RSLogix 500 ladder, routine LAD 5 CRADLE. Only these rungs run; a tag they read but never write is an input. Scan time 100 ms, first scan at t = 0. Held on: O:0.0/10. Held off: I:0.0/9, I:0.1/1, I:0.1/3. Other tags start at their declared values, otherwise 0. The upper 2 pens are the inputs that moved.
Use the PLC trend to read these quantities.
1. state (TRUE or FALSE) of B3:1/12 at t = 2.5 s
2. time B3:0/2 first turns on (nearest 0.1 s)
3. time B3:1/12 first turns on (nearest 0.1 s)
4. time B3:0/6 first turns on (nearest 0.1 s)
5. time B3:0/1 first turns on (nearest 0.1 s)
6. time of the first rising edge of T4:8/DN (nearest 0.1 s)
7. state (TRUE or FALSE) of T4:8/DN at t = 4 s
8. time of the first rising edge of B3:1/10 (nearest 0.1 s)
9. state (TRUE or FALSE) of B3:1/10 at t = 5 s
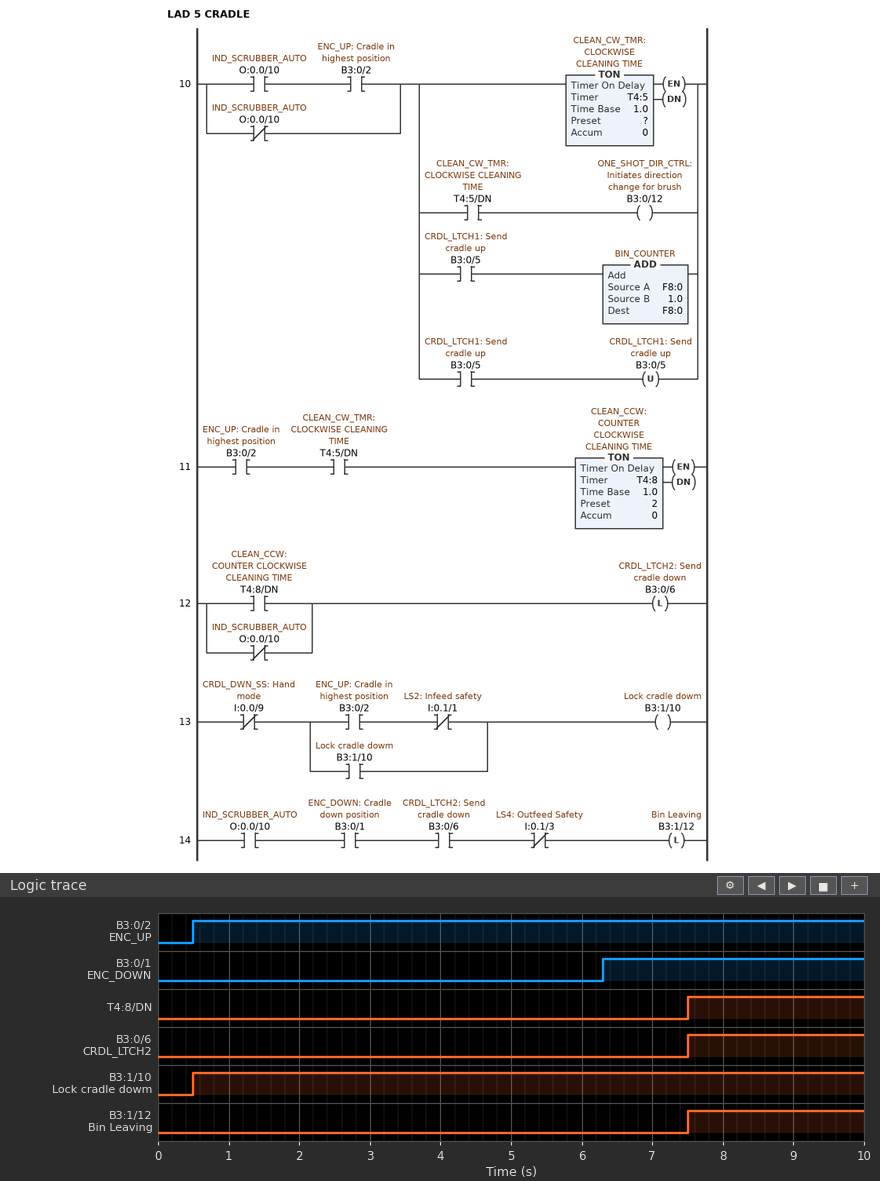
FALSE
0.5 s
7.5 s
7.5 s
6.3 s
7.5 s
FALSE
0.5 s
TRUE
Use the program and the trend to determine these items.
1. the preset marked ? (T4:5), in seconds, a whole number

5 s
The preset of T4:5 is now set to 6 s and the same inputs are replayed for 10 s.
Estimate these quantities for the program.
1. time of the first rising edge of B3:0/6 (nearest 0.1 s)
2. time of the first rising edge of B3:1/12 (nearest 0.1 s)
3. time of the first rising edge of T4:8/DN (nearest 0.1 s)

8.5 s
8.5 s
8.5 s
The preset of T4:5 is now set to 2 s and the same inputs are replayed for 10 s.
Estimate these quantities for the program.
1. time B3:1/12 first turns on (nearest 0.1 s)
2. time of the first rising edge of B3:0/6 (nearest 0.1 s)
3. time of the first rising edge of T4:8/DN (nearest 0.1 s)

6.3 s
4.5 s
4.5 s
